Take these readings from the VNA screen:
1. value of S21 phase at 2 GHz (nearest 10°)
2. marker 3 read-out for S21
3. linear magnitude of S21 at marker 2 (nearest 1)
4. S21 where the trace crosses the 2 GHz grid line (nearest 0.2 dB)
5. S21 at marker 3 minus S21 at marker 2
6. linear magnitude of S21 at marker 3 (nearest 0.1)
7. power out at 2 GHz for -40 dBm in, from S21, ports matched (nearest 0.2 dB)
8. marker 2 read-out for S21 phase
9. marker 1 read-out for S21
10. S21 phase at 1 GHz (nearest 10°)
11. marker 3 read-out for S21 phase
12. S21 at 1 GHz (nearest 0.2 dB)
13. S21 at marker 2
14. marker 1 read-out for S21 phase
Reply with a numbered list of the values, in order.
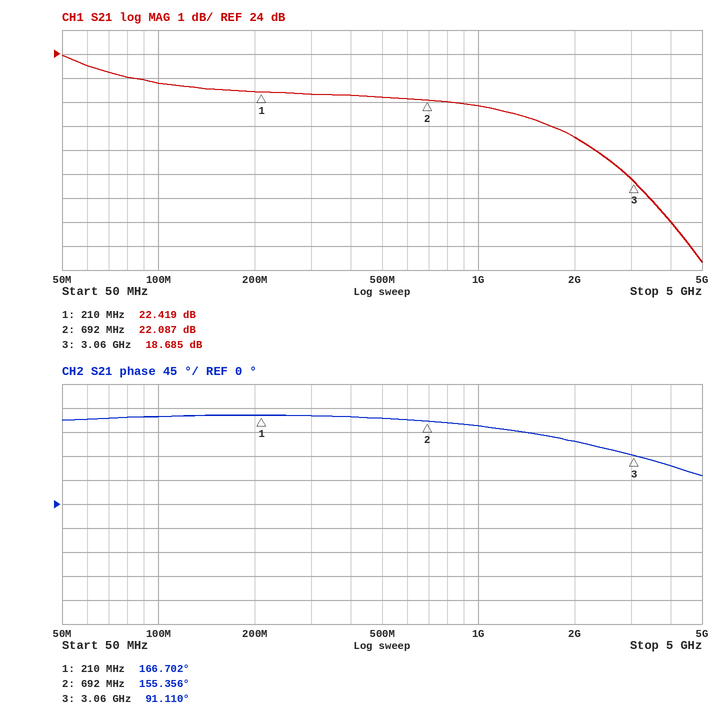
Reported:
1. 120°
2. 18.685 dB
3. 13
4. 20.6 dB
5. -3.402 dB
6. 8.6
7. -19.4 dBm
8. 155.356°
9. 22.419 dB
10. 150°
11. 91.110°
12. 21.8 dB
13. 22.087 dB
14. 166.702°
